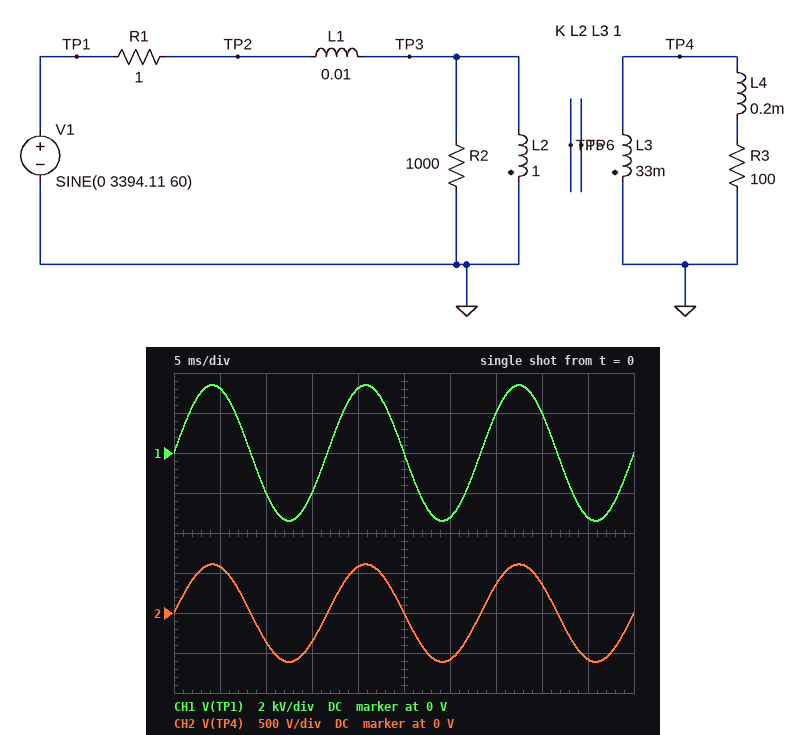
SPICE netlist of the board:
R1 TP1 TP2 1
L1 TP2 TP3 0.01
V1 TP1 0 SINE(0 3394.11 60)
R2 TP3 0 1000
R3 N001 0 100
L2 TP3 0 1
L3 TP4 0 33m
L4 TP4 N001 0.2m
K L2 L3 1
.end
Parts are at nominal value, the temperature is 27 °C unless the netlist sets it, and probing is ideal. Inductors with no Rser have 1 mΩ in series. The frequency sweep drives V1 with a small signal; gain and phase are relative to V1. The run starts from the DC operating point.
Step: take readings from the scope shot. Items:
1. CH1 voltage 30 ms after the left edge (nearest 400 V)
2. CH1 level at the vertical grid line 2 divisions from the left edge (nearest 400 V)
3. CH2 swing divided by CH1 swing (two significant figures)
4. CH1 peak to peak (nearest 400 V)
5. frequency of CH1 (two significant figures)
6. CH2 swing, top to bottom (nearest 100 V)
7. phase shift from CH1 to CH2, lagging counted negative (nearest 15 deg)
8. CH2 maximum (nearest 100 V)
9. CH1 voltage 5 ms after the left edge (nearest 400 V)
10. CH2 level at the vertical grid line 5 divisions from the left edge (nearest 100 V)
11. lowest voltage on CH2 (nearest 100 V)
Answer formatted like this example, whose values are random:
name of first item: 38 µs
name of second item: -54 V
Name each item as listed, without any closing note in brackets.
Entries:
CH1 voltage 30 ms after the left edge: -3.2 kV
CH1 level at the vertical grid line 2 divisions from the left edge: -2.0 kV
CH2 swing divided by CH1 swing: 0.18
CH1 peak to peak: 6.8 kV
frequency of CH1: 60 Hz
CH2 swing, top to bottom: 1.2 kV
phase shift from CH1 to CH2, lagging counted negative: 0 deg
CH2 maximum: 600 V
CH1 voltage 5 ms after the left edge: 3.2 kV
CH2 level at the vertical grid line 5 divisions from the left edge: 0 V
lowest voltage on CH2: -600 V
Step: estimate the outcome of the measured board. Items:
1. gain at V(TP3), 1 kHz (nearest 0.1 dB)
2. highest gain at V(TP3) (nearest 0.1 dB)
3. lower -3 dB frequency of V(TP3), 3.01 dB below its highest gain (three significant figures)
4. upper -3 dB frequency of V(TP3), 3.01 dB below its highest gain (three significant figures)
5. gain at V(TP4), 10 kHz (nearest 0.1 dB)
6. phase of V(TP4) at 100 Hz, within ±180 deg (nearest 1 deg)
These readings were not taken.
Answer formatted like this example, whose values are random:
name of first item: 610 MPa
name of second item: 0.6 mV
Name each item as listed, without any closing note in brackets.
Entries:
gain at V(TP3), 1 kHz: -0.1 dB
highest gain at V(TP3): -0.1 dB
lower -3 dB frequency of V(TP3), 3.01 dB below its highest gain: 158 mHz
upper -3 dB frequency of V(TP3), 3.01 dB below its highest gain: 11.7 kHz
gain at V(TP4), 10 kHz: -17.3 dB
phase of V(TP4) at 100 Hz, within ±180 deg: 0 deg
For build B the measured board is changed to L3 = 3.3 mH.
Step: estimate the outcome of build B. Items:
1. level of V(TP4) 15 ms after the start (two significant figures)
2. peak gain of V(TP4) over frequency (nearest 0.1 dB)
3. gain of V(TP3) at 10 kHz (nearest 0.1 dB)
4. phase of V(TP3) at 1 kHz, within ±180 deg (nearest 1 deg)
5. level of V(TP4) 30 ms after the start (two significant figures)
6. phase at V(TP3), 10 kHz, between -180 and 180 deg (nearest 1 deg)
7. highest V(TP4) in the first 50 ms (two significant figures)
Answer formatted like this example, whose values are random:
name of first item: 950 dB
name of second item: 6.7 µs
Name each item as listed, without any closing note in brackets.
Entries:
level of V(TP4) 15 ms after the start: -110 V
peak gain of V(TP4) over frequency: -24.9 dB
gain of V(TP3) at 10 kHz: -1.6 dB
phase of V(TP3) at 1 kHz, within ±180 deg: -4 deg
level of V(TP4) 30 ms after the start: -180 V
phase at V(TP3), 10 kHz, between -180 and 180 deg: -33 deg
highest V(TP4) in the first 50 ms: 190 V
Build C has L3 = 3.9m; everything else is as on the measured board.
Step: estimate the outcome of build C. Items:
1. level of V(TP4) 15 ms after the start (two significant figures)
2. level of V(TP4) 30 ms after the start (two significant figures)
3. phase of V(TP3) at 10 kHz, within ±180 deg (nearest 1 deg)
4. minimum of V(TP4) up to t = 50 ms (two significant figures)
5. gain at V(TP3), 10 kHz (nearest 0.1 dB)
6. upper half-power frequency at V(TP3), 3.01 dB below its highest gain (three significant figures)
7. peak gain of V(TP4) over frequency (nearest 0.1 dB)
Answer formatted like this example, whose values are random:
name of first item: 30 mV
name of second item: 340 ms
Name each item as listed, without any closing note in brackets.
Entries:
level of V(TP4) 15 ms after the start: -120 V
level of V(TP4) 30 ms after the start: -200 V
phase of V(TP3) at 10 kHz, within ±180 deg: -33 deg
minimum of V(TP4) up to t = 50 ms: -210 V
gain at V(TP3), 10 kHz: -1.6 dB
upper half-power frequency at V(TP3), 3.01 dB below its highest gain: 15.4 kHz
peak gain of V(TP4) over frequency: -24.2 dB
